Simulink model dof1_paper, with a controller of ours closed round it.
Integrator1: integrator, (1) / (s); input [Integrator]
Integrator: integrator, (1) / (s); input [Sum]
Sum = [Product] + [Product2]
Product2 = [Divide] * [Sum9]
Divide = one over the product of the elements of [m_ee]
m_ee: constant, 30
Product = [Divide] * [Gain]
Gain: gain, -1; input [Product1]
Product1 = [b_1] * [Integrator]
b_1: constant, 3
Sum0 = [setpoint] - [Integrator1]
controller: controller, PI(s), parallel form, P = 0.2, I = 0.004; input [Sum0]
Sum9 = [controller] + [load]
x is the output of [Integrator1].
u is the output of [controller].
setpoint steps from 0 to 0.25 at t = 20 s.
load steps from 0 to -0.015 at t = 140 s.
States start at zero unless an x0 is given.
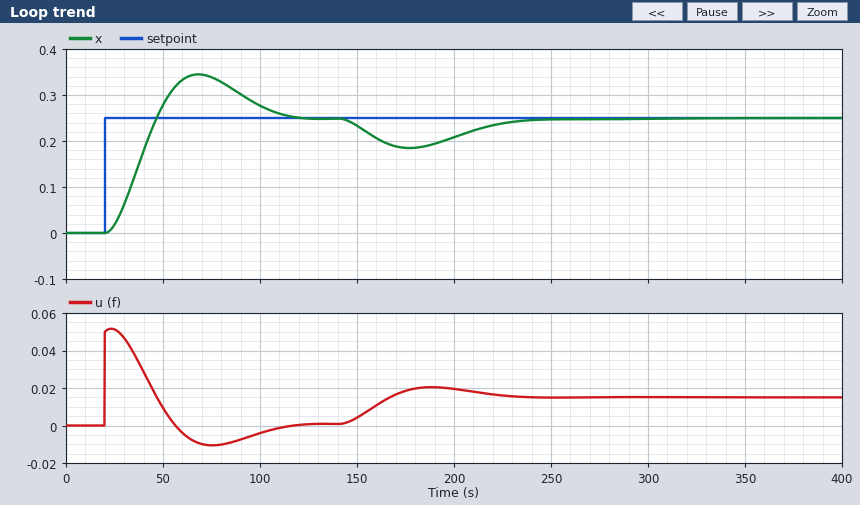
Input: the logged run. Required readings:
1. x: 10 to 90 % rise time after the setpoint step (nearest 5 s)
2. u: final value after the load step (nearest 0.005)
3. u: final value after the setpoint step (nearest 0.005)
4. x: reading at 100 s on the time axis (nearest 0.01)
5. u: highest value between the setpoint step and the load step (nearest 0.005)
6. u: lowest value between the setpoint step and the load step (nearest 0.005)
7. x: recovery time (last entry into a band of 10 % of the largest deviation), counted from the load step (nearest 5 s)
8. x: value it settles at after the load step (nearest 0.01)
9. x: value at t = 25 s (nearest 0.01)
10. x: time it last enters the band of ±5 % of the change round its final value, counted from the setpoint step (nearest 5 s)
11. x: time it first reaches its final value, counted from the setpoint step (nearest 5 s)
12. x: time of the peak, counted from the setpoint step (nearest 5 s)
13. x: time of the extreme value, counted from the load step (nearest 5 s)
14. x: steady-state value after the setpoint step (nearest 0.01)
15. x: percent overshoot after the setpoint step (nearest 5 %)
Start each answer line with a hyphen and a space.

- 20 s
- 0.015
- 0.000
- 0.28
- 0.050
- -0.010
- 95 s
- 0.25
- 0.02
- 90 s
- 25 s
- 50 s
- 35 s
- 0.25
- 40 %
